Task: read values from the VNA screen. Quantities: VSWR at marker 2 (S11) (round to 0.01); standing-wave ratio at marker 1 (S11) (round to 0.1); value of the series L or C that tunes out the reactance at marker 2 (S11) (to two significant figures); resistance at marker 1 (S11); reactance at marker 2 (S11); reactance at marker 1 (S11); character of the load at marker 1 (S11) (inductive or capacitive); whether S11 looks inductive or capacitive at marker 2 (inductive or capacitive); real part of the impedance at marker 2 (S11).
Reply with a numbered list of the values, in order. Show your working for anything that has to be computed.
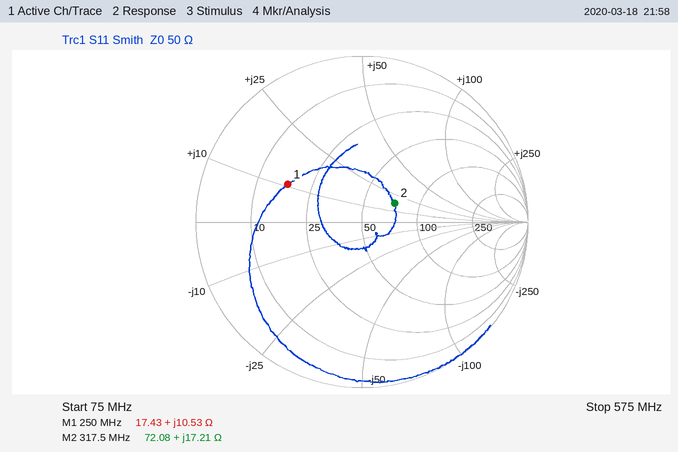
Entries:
1. 1.59
2. 3.0
3. C = 1/(2π × 317.5 MHz × 17.21 Ω) ≈ 29 pF
4. 17.43 Ω
5. +17.21 Ω
6. +10.53 Ω
7. inductive
8. inductive
9. 72.08 Ω
